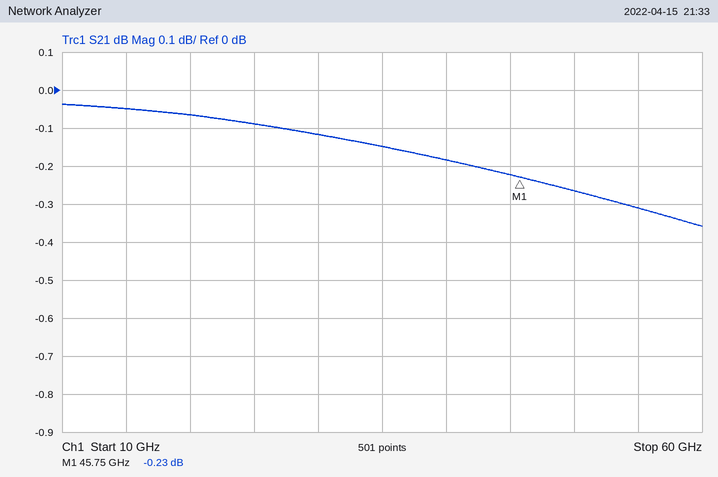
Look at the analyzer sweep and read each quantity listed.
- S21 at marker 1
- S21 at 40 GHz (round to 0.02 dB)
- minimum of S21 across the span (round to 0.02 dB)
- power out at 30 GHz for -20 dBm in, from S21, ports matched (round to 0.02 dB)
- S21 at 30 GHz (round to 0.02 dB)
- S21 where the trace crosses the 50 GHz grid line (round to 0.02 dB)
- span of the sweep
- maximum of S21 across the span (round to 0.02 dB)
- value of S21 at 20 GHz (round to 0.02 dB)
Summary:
-0.23 dB
-0.18 dB
-0.36 dB
-20.12 dBm
-0.12 dB
-0.26 dB
50 GHz
-0.04 dB
-0.06 dB
